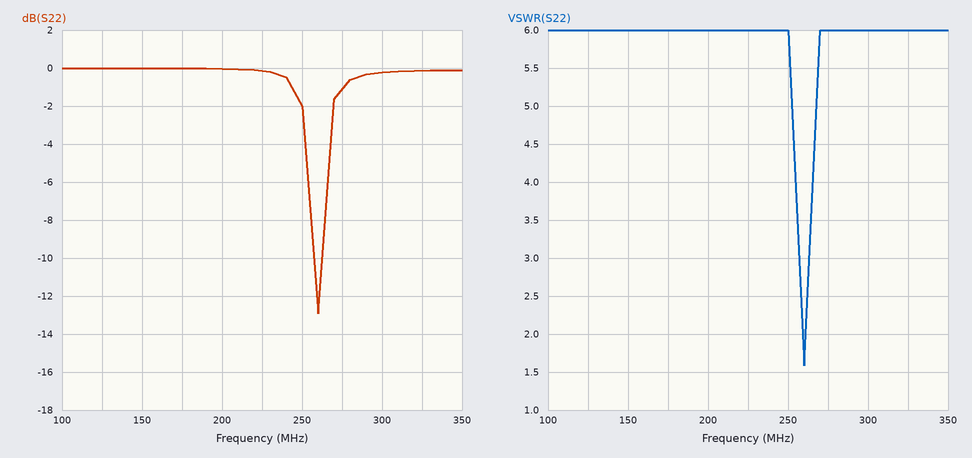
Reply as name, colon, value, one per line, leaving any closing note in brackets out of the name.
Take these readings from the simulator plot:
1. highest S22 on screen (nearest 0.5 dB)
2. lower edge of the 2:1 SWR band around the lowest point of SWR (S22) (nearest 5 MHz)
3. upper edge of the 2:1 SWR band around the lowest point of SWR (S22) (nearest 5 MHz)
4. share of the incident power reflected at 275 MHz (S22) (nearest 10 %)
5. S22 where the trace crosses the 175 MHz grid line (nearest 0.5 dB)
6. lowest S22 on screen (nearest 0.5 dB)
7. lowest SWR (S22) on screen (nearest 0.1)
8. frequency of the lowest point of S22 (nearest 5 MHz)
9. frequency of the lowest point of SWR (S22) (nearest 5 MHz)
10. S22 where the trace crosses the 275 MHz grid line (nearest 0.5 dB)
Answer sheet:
highest S22 on screen: 0.0 dB
lower edge of the 2:1 SWR band around the lowest point of SWR (S22): 260 MHz
upper edge of the 2:1 SWR band around the lowest point of SWR (S22): 260 MHz
share of the incident power reflected at 275 MHz (S22): 80 %
S22 where the trace crosses the 175 MHz grid line: 0.0 dB
lowest S22 on screen: -13.0 dB
lowest SWR (S22) on screen: 1.6
frequency of the lowest point of S22: 260 MHz
frequency of the lowest point of SWR (S22): 260 MHz
S22 where the trace crosses the 275 MHz grid line: -1.0 dB
